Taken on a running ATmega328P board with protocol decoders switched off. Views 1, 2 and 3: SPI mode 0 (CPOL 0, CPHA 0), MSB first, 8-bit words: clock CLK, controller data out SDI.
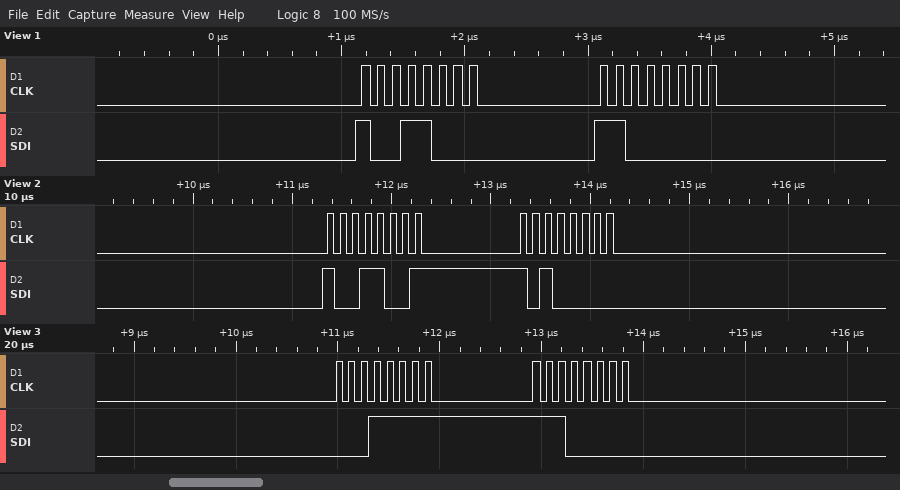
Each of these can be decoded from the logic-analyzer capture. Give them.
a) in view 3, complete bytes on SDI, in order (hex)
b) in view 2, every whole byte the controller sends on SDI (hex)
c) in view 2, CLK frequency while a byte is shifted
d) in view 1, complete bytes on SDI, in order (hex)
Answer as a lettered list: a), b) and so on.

a) 0x1F 0xE0
b) 99 A0
c) 8 MHz
d) 98 C0
